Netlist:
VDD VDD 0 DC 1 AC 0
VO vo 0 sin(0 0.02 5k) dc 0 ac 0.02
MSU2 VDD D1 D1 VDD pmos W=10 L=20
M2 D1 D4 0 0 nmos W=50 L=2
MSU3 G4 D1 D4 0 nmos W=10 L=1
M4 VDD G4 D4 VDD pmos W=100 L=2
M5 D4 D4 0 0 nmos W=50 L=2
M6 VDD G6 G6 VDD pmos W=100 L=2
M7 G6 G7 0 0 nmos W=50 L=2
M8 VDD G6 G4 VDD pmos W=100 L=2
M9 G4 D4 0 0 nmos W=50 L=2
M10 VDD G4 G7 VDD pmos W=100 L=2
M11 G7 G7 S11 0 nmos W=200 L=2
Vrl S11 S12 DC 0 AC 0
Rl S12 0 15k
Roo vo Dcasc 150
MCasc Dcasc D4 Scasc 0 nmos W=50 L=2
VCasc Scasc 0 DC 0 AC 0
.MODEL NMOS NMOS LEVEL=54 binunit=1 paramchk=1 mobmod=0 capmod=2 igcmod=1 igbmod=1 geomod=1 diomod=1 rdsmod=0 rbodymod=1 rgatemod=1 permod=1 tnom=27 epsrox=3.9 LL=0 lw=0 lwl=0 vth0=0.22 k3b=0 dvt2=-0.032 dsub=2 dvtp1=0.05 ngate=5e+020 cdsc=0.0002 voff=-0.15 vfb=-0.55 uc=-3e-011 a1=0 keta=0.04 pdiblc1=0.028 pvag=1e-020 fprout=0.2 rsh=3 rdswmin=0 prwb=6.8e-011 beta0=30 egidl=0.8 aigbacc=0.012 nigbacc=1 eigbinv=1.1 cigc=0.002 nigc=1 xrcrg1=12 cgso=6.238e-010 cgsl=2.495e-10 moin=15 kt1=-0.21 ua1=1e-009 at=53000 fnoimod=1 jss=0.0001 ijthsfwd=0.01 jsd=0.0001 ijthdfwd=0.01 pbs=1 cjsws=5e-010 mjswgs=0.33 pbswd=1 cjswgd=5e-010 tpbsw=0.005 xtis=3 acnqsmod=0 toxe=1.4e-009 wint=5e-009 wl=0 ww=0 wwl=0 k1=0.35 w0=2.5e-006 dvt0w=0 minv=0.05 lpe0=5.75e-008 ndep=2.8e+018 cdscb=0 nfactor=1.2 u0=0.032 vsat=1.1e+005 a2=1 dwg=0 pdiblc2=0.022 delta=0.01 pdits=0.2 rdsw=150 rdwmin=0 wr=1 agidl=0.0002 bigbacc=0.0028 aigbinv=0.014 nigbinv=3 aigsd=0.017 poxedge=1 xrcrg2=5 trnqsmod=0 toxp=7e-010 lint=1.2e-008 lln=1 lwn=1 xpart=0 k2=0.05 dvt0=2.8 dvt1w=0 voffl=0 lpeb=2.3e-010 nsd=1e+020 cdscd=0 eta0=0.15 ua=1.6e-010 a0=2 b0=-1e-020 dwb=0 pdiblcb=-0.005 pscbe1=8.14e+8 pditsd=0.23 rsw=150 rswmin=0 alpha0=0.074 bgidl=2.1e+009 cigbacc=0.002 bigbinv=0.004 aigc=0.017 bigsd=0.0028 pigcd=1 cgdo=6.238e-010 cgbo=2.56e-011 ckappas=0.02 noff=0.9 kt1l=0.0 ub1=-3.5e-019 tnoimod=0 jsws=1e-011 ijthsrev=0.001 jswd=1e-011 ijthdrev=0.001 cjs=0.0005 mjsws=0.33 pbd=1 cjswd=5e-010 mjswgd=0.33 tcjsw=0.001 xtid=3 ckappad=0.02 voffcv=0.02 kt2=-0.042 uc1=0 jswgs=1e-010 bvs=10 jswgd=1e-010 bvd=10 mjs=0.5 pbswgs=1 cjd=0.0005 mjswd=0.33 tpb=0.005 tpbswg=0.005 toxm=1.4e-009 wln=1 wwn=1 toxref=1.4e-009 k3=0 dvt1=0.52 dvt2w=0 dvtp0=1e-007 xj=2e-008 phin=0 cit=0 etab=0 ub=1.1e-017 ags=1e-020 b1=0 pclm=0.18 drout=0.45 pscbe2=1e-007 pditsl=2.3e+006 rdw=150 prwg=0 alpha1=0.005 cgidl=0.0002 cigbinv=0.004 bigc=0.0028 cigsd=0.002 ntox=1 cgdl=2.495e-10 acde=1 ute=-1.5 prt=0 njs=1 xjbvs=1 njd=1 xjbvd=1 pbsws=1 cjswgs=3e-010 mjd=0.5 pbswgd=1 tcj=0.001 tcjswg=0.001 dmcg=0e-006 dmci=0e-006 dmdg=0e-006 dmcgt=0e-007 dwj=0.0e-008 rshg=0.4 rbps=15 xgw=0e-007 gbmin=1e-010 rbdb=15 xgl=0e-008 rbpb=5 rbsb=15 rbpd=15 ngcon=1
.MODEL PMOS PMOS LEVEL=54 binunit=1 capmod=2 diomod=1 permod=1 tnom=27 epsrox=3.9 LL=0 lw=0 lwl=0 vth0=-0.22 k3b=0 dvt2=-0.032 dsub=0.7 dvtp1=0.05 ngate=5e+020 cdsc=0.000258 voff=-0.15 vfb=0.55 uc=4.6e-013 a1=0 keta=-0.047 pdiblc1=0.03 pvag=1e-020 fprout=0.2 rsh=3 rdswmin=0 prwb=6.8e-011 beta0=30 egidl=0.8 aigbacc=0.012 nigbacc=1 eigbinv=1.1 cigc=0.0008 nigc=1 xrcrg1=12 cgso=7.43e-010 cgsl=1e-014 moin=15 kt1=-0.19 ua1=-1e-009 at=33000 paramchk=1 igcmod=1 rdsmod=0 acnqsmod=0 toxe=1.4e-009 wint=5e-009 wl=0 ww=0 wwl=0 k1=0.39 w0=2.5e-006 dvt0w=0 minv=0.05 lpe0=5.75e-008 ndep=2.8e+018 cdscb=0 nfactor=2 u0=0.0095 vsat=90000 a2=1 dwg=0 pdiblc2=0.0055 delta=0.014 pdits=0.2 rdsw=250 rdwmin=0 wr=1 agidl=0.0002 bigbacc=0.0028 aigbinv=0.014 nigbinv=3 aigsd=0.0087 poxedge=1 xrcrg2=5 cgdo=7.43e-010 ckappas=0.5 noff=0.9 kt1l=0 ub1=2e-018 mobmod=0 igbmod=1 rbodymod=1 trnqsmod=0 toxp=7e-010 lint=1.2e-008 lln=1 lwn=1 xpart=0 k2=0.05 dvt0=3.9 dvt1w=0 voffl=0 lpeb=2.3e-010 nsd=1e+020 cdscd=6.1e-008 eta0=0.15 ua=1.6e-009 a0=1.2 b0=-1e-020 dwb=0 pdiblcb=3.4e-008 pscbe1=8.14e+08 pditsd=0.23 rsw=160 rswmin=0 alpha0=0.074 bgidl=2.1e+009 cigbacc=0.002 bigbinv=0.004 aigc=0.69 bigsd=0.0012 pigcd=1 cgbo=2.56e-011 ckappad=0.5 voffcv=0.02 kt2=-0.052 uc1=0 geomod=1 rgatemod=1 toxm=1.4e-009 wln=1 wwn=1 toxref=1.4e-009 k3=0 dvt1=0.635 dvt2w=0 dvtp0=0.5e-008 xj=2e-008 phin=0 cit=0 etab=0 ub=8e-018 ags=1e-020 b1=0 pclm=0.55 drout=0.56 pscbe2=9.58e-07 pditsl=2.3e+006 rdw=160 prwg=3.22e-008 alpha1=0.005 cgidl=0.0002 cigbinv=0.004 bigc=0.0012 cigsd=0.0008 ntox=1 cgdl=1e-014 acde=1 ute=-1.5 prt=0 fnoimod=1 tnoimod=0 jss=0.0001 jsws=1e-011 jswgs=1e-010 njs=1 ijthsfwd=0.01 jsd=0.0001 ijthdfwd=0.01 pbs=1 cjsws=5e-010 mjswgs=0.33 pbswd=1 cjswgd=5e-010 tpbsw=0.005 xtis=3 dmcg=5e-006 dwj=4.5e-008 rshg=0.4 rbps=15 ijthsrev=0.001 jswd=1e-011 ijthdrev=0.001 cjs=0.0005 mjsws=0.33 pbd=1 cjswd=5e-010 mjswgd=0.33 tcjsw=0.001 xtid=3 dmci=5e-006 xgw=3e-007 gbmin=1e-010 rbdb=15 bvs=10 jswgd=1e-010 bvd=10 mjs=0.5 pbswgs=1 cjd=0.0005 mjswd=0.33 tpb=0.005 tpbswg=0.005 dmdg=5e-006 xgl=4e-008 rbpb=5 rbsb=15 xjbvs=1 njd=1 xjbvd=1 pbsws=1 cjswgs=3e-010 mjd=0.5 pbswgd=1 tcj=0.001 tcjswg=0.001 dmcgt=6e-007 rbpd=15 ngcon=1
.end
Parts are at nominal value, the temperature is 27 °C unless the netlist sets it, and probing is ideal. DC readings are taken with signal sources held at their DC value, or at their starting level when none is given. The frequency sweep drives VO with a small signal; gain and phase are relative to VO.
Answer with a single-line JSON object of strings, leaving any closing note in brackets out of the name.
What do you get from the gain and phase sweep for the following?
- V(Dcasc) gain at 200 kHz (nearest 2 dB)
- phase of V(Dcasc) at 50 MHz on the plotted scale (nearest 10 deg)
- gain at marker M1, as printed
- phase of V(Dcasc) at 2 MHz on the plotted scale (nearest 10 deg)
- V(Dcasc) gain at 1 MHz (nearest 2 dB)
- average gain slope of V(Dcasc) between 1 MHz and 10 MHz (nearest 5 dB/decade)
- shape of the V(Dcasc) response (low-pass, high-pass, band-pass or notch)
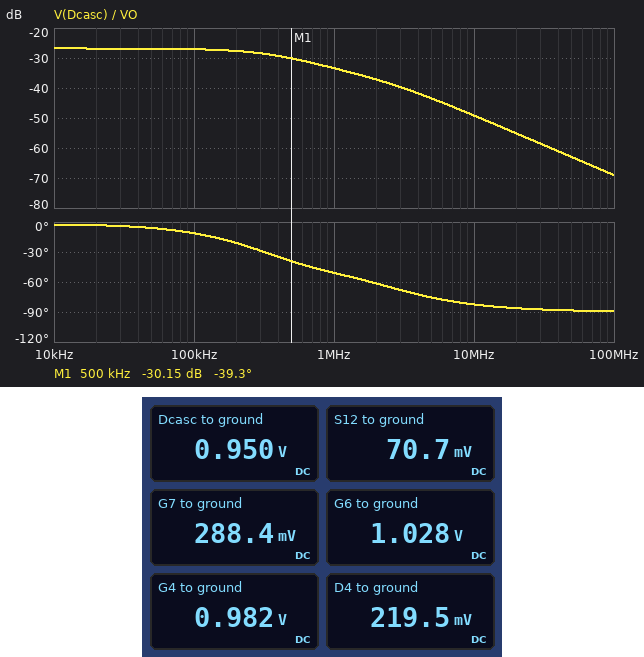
{"V(Dcasc) gain at 200 kHz": "-28 dB", "phase of V(Dcasc) at 50 MHz on the plotted scale": "-90 deg", "gain at marker M1, as printed": "-30.15 dB", "phase of V(Dcasc) at 2 MHz on the plotted scale": "-60 deg", "V(Dcasc) gain at 1 MHz": "-34 dB", "average gain slope of V(Dcasc) between 1 MHz and 10 MHz": "-15 dB/decade", "shape of the V(Dcasc) response": "low-pass"}
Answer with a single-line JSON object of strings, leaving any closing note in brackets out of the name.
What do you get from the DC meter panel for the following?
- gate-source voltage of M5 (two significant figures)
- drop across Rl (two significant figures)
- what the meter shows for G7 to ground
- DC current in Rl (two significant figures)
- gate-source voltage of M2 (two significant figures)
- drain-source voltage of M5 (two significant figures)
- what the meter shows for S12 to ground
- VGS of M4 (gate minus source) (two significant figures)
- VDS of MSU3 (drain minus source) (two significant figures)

{"gate-source voltage of M5": "220 mV", "drop across Rl": "71 mV", "what the meter shows for G7 to ground": "288.4 mV", "DC current in Rl": "4.7 µA", "gate-source voltage of M2": "220 mV", "drain-source voltage of M5": "220 mV", "what the meter shows for S12 to ground": "70.7 mV", "VGS of M4 (gate minus source)": "760 mV", "VDS of MSU3 (drain minus source)": "760 mV"}
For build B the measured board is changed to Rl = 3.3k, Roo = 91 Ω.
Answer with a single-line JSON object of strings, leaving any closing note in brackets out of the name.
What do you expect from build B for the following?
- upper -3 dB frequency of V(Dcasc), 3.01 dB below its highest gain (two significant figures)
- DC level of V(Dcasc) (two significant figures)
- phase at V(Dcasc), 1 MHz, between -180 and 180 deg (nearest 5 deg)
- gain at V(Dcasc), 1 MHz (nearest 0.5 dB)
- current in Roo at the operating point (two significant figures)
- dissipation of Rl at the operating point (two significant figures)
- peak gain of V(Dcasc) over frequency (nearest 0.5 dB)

{"upper -3 dB frequency of V(Dcasc), 3.01 dB below its highest gain": "290 kHz", "DC level of V(Dcasc)": "920 mV", "phase at V(Dcasc), 1 MHz, between -180 and 180 deg": "-55 deg", "gain at V(Dcasc), 1 MHz": "-29.0 dB", "current in Roo at the operating point": "10 mA", "dissipation of Rl at the operating point": "1.5 µW", "peak gain of V(Dcasc) over frequency": "-20.5 dB"}
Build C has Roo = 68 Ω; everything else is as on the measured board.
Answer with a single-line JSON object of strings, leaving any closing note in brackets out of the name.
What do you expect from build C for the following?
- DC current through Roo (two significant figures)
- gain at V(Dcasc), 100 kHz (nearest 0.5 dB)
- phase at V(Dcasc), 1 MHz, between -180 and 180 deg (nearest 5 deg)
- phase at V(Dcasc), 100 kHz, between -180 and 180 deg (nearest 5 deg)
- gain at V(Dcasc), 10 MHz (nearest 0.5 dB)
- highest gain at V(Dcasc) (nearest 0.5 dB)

{"DC current through Roo": "13 mA", "gain at V(Dcasc), 100 kHz": "-18.5 dB", "phase at V(Dcasc), 1 MHz, between -180 and 180 deg": "-55 deg", "phase at V(Dcasc), 100 kHz, between -180 and 180 deg": "-15 deg", "gain at V(Dcasc), 10 MHz": "-42.5 dB", "highest gain at V(Dcasc)": "-17.0 dB"}
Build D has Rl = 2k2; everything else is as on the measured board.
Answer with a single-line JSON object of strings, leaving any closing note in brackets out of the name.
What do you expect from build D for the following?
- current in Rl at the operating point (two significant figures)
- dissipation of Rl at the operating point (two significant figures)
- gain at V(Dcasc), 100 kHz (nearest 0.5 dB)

{"current in Rl at the operating point": "32 µA", "dissipation of Rl at the operating point": "2.3 µW", "gain at V(Dcasc), 100 kHz": "-27.0 dB"}
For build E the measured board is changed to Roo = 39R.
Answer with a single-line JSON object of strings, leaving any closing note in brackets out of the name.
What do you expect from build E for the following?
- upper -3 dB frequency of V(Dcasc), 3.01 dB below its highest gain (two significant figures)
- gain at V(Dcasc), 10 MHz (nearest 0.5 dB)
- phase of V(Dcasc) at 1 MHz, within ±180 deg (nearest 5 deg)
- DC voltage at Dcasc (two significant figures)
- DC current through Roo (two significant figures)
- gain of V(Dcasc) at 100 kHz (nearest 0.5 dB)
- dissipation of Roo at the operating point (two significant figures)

{"upper -3 dB frequency of V(Dcasc), 3.01 dB below its highest gain": "210 kHz", "gain at V(Dcasc), 10 MHz": "-38.5 dB", "phase of V(Dcasc) at 1 MHz, within ±180 deg": "-60 deg", "DC voltage at Dcasc": "790 mV", "DC current through Roo": "20 mA", "gain of V(Dcasc) at 100 kHz": "-11.5 dB", "dissipation of Roo at the operating point": "16 mW"}
